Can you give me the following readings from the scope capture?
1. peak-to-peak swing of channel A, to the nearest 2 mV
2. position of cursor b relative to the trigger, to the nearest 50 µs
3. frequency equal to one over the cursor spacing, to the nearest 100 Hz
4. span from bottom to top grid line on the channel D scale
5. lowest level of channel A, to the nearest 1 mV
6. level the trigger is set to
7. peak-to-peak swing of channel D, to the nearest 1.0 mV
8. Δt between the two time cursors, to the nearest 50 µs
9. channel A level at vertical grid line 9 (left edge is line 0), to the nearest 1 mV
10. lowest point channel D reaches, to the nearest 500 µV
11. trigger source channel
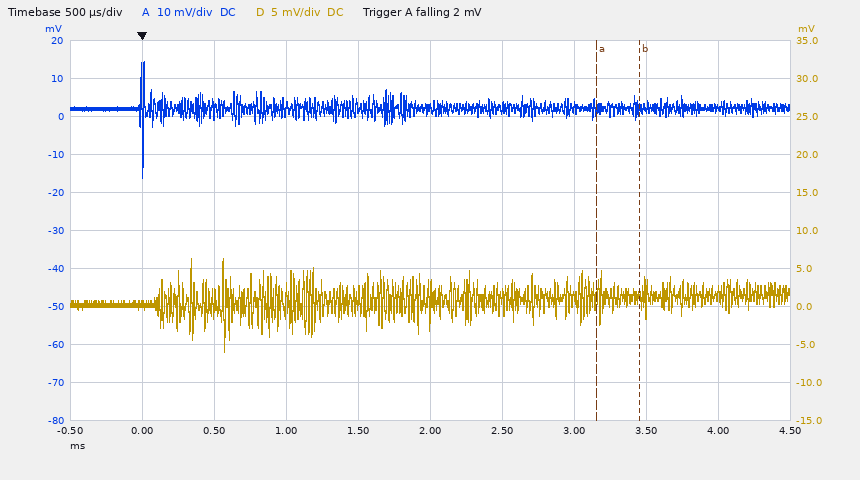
30 mV
+3.45 ms
3.3 kHz
50 mV
-16 mV
2 mV
12.0 mV
300 µs
2 mV
-6.0 mV
channel A
